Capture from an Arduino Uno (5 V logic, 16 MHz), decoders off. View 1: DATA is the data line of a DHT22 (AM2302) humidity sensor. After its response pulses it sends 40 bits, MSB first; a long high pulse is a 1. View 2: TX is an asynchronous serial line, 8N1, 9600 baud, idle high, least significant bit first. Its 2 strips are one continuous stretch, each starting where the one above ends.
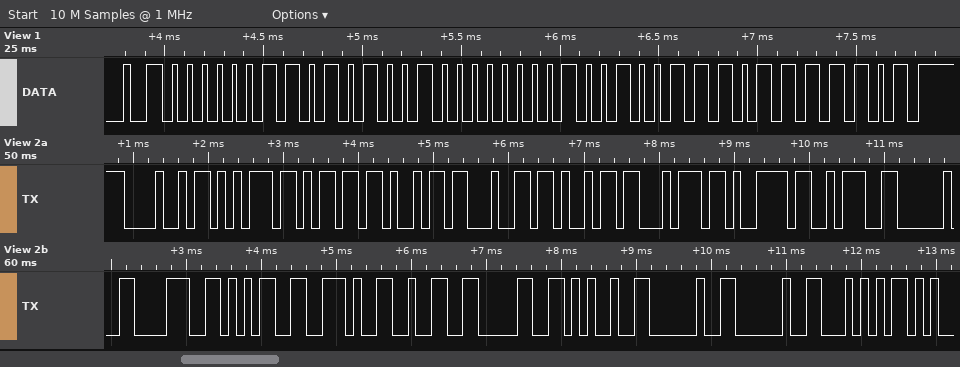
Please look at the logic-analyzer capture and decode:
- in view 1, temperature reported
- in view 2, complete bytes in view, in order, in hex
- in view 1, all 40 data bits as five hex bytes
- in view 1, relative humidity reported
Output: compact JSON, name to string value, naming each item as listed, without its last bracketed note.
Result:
{"in view 1, temperature reported": "29.5 °C", "in view 2, complete bytes in view, in order, in hex": "0x48 0x75 0x6D 0x69 0x64 0x69 0x74 0x79 0x3A 0x20 0x38 0x35 0x2E 0x32 0x30 0x25 0x20 0x20 0x54", "in view 1, all 40 data bits as five hex bytes": "03 52 01 27 7D", "in view 1, relative humidity reported": "85.0 %"}
